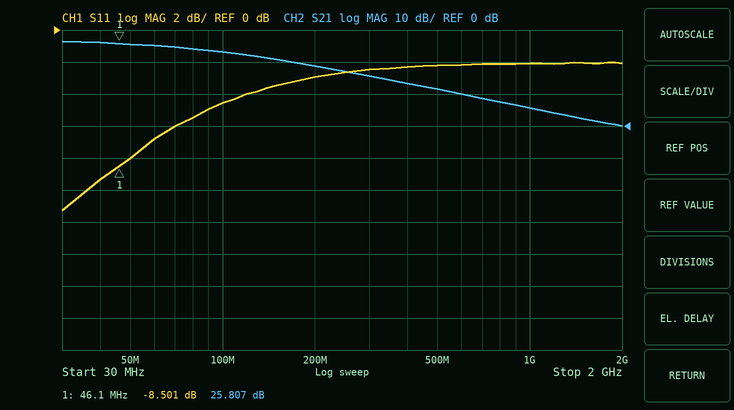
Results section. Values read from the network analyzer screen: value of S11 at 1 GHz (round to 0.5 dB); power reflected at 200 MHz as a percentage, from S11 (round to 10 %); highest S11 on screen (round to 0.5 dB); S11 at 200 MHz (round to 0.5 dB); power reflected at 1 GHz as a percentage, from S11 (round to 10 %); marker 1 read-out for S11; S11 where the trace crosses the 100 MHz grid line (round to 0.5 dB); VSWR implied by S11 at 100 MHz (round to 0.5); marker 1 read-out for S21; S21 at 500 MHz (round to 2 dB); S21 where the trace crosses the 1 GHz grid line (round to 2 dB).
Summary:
-2.0 dB
50 %
-2.0 dB
-3.0 dB
60 %
-8.501 dB
-4.5 dB
4.0
25.807 dB
12 dB
6 dB
